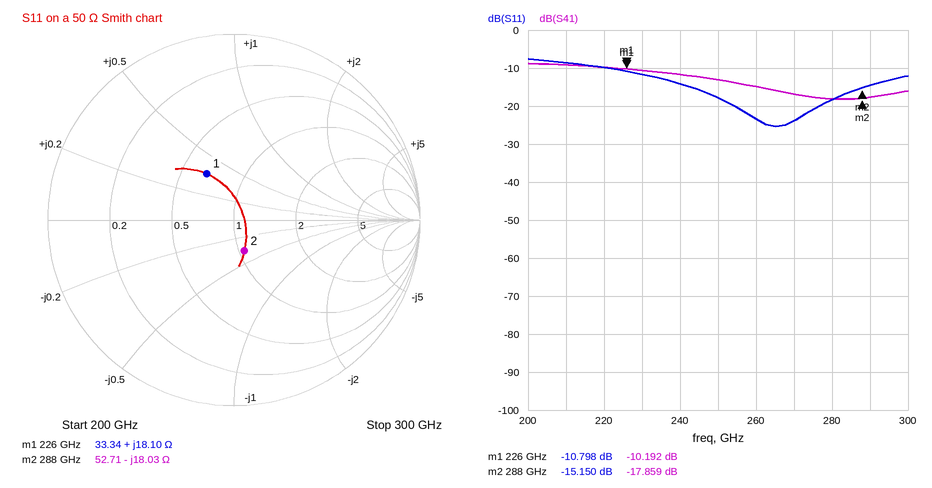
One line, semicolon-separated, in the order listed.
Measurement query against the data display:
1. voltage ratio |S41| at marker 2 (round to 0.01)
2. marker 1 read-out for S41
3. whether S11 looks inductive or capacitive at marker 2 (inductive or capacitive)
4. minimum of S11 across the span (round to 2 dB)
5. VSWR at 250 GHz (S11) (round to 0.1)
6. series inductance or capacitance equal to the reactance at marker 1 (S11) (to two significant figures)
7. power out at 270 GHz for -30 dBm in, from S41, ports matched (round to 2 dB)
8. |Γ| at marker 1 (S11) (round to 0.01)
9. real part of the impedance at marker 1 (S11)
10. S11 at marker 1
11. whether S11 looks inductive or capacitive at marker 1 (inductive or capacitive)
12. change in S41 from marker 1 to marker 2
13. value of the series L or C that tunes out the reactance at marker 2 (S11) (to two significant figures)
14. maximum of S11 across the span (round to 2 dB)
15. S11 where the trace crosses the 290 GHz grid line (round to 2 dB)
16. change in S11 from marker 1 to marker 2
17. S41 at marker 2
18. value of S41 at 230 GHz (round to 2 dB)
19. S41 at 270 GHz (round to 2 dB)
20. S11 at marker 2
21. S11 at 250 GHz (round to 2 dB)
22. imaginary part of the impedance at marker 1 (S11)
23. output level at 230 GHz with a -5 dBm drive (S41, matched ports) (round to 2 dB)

0.13; -10.192 dB; capacitive; -26 dB; 1.3; 13 pH; -46 dBm; 0.29; 33.34 Ω; -10.798 dB; inductive; -7.667 dB; 10.0 pH; -8 dB; -14 dB; -4.352 dB; -17.859 dB; -10 dB; -16 dB; -15.150 dB; -18 dB; +18.10 Ω; -16 dBm
